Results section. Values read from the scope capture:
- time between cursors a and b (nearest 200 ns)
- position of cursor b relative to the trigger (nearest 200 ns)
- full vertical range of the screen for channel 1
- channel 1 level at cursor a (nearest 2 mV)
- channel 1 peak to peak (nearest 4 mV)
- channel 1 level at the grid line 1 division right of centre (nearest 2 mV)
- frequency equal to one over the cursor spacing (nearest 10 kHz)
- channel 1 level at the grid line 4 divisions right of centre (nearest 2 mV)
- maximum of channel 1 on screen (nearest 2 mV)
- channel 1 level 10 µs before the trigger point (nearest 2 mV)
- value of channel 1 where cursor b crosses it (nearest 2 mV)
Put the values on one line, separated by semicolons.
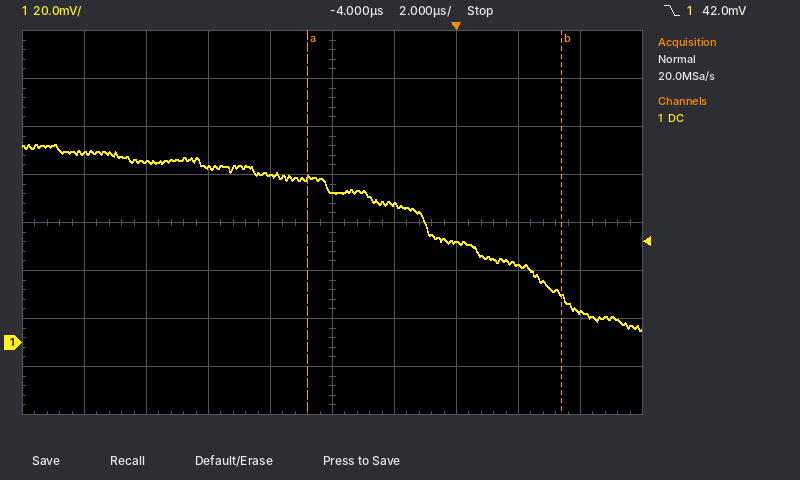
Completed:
8.2 µs; +3.4 µs; 160 mV; 68 mV; 76 mV; 58 mV; 120 kHz; 12 mV; 82 mV; 76 mV; 20 mV
